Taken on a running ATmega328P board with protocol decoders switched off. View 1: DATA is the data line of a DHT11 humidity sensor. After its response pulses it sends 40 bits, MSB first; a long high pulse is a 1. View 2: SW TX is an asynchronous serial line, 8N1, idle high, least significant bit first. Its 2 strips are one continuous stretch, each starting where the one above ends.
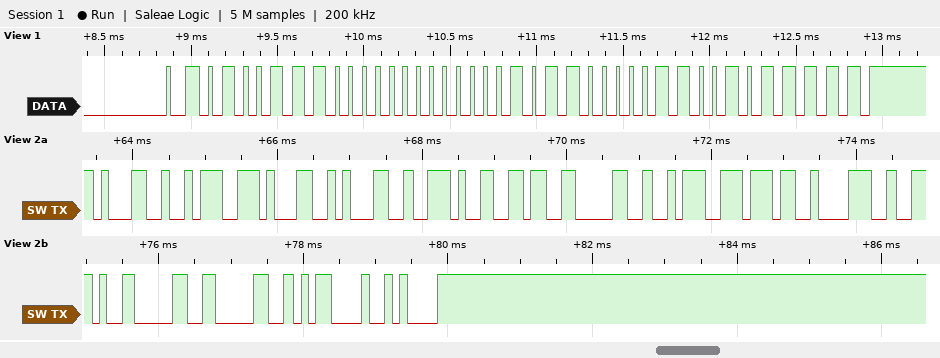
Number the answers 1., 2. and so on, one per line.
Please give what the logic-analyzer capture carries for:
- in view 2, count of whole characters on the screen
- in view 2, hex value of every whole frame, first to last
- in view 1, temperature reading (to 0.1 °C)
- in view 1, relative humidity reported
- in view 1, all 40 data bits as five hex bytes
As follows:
1. 15
2. 0x31 0x3A 0x31 0x31 0x2E 0x36 0x30 0x3A 0x37 0x38 0x2E 0x30 0x30 0x0D 0x0A
3. 11.6 °C
4. 78 %
5. 4E 00 0B 06 5F
